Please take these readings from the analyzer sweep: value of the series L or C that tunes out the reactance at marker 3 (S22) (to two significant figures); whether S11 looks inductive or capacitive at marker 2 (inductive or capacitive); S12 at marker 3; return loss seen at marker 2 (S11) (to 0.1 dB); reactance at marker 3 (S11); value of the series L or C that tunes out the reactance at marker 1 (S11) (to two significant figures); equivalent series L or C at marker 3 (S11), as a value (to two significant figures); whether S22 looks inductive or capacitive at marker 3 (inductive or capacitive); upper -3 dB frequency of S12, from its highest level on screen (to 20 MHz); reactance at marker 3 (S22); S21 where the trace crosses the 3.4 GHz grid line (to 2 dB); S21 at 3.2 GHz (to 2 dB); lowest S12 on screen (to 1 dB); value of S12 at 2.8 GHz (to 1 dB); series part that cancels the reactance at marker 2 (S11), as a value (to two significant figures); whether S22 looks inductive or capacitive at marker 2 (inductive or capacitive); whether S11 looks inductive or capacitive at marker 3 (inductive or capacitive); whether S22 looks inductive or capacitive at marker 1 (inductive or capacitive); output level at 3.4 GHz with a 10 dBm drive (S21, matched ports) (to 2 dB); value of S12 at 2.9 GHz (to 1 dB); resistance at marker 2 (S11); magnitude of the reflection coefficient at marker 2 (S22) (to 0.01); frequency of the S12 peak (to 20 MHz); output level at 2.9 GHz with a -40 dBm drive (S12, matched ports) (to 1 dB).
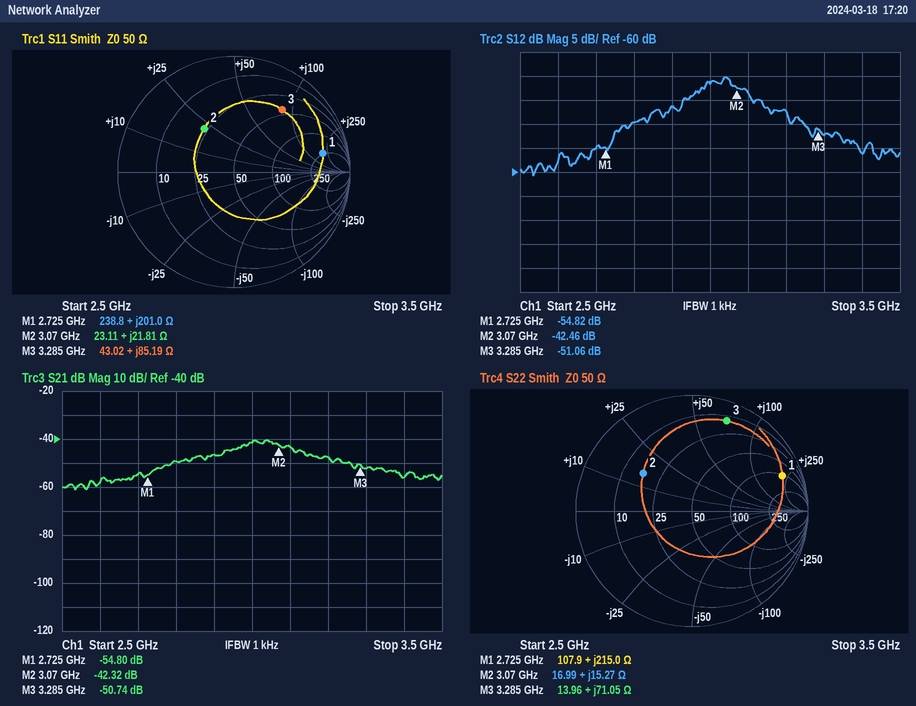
680 fF
inductive
-51.06 dB
6.9 dB
+85.19 Ω
290 fF
4.1 nH
inductive
3.10 GHz
+71.05 Ω
-56 dB
-48 dB
-61 dB
-50 dB
2.4 pF
inductive
inductive
inductive
-46 dBm
-46 dB
23.11 Ω
0.53
3.04 GHz
-86 dBm
